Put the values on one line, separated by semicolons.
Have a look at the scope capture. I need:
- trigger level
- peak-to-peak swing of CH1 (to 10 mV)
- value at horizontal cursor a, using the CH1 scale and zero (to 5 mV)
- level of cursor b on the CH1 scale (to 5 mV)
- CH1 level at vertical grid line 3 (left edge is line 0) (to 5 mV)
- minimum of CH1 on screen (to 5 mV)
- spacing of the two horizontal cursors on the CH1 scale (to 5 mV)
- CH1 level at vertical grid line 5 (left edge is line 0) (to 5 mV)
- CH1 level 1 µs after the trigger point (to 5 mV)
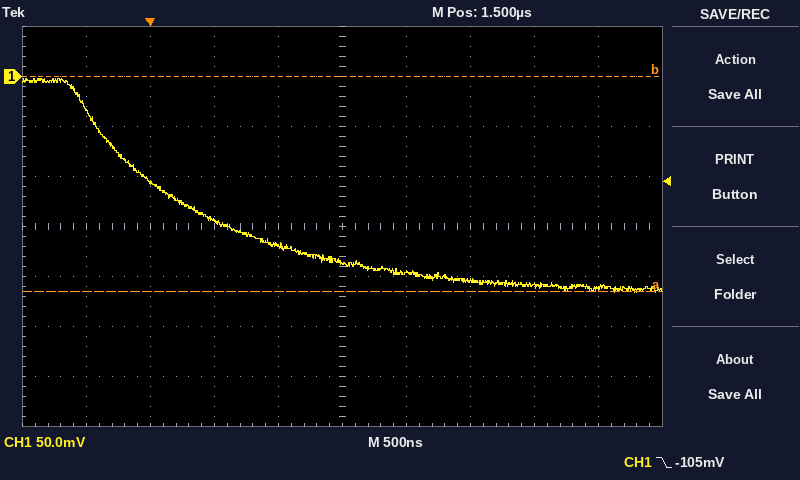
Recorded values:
-105 mV; 210 mV; -215 mV; 0 mV; -145 mV; -215 mV; 215 mV; -185 mV; -170 mV
